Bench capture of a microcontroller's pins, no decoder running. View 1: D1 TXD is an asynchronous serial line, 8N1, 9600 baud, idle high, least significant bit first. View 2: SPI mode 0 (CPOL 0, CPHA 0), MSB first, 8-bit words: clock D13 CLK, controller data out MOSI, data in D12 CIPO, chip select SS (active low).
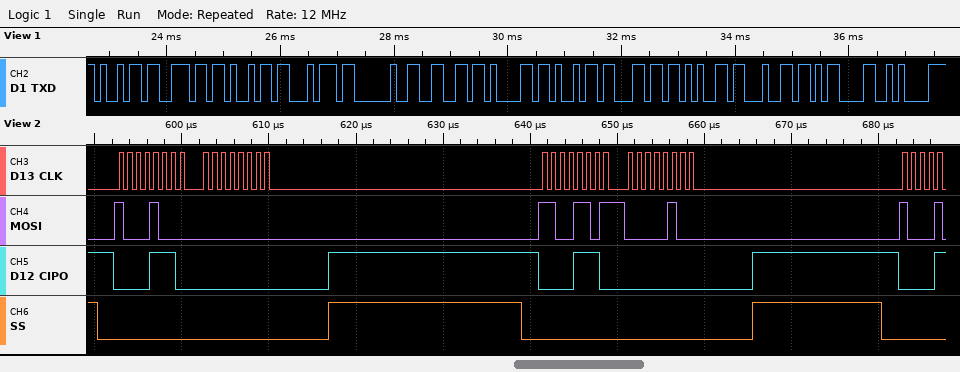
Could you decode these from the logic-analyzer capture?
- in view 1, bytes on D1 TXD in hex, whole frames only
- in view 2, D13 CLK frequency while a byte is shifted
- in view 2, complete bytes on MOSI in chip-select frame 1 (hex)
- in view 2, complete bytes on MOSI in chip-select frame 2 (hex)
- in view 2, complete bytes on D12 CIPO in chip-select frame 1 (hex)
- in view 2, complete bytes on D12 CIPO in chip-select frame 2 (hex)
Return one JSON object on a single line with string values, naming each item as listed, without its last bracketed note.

{"in view 1, bytes on D1 TXD in hex, whole frames only": "69 6E 69 74 20 66 61 69 6C 65 64 0D 0A", "in view 2, D13 CLK frequency while a byte is shifted": "1 MHz", "in view 2, complete bytes on MOSI in chip-select frame 1": "88 00", "in view 2, complete bytes on MOSI in chip-select frame 2": "CD 04", "in view 2, complete bytes on D12 CIPO in chip-select frame 1": "0E 00", "in view 2, complete bytes on D12 CIPO in chip-select frame 2": "0E 00"}
